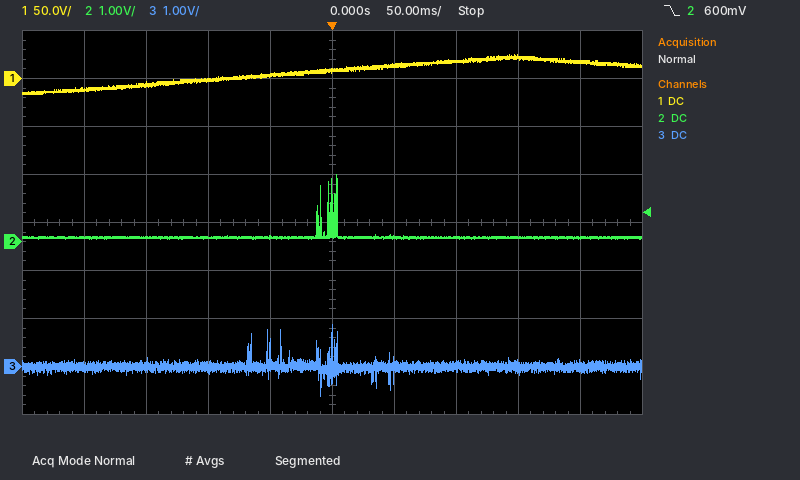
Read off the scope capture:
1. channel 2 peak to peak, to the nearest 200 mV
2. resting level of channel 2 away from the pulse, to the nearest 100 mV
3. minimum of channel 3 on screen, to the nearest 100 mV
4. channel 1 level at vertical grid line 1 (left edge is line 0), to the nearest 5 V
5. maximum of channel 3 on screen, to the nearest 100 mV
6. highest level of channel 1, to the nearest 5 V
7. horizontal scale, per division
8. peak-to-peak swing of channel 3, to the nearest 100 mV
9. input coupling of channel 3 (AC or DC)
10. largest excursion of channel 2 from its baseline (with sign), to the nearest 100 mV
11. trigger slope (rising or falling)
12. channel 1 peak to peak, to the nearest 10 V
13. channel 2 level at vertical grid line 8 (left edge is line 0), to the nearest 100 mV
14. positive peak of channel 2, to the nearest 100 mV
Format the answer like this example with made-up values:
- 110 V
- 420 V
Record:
- 1.4 V
- 100 mV
- -600 mV
- -10 V
- 900 mV
- 25 V
- 50 ms
- 1.5 V
- DC
- +1.3 V
- falling
- 40 V
- 100 mV
- 1.4 V
